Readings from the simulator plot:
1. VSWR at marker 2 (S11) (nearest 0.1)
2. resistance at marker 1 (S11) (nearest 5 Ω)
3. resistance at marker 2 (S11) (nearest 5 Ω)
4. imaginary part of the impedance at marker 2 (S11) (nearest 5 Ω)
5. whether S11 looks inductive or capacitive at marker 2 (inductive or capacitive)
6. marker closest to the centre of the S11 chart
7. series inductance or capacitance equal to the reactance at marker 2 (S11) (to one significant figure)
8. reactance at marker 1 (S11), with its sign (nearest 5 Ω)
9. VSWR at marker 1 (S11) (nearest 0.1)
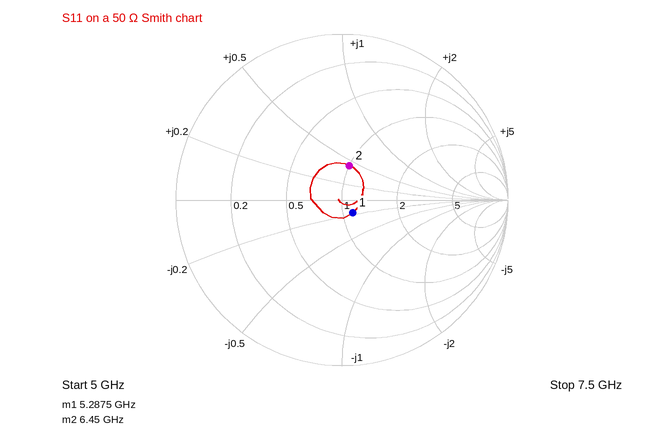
1.5
55 Ω
50 Ω
+20 Ω
inductive
marker 1
500 pH
-10 Ω
1.2
